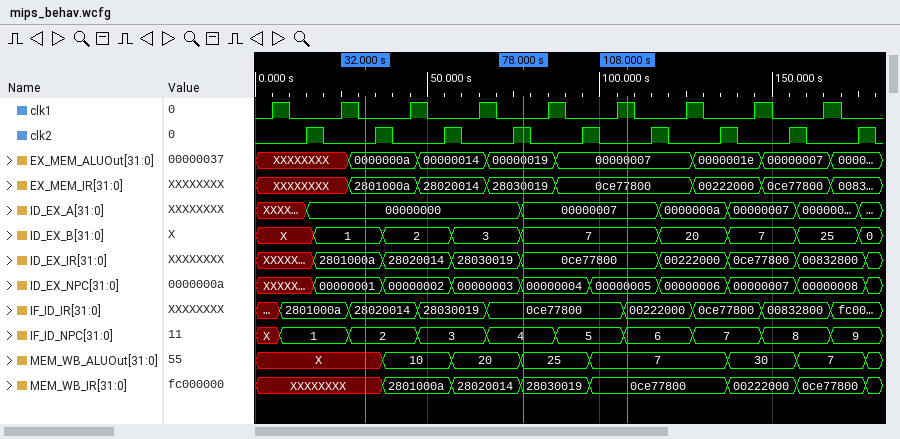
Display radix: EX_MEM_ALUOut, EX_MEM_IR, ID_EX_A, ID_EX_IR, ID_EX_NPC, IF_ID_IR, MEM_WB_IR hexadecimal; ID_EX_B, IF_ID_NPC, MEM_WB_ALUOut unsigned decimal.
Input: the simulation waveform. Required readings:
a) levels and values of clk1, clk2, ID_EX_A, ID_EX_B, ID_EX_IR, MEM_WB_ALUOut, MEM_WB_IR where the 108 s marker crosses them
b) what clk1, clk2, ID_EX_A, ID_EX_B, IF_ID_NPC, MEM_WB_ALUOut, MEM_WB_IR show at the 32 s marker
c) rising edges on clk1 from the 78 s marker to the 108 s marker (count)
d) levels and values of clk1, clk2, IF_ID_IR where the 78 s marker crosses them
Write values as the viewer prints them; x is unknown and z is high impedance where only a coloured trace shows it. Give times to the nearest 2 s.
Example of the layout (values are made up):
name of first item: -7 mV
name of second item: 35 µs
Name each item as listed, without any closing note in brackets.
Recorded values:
levels and values of clk1, clk2, ID_EX_A, ID_EX_B, ID_EX_IR, MEM_WB_ALUOut, MEM_WB_IR where the 108 s marker crosses them: clk1=1, clk2=0, ID_EX_A=00000007, ID_EX_B=7, ID_EX_IR=0ce77800, MEM_WB_ALUOut=7, MEM_WB_IR=0ce77800
what clk1, clk2, ID_EX_A, ID_EX_B, IF_ID_NPC, MEM_WB_ALUOut, MEM_WB_IR show at the 32 s marker: clk1=0, clk2=0, ID_EX_A=00000000, ID_EX_B=1, IF_ID_NPC=2, MEM_WB_ALUOut=X, MEM_WB_IR=XXXXXXXX
rising edges on clk1 from the 78 s marker to the 108 s marker: 2
levels and values of clk1, clk2, IF_ID_IR where the 78 s marker crosses them: clk1=0, clk2=1, IF_ID_IR=0ce77800
